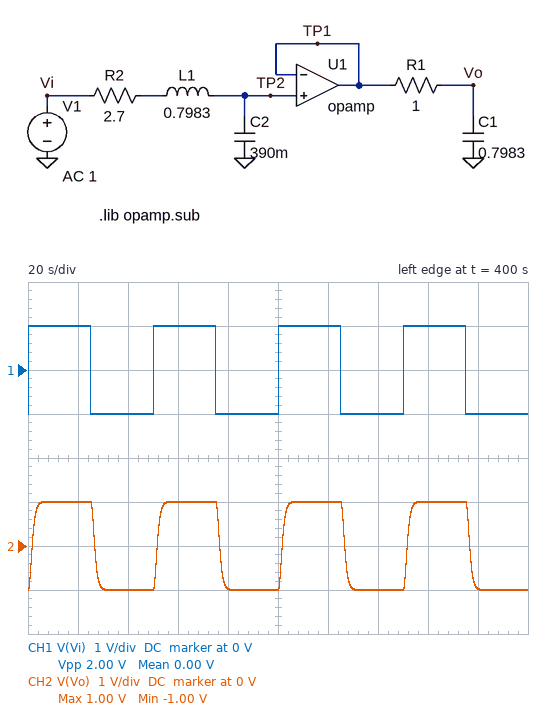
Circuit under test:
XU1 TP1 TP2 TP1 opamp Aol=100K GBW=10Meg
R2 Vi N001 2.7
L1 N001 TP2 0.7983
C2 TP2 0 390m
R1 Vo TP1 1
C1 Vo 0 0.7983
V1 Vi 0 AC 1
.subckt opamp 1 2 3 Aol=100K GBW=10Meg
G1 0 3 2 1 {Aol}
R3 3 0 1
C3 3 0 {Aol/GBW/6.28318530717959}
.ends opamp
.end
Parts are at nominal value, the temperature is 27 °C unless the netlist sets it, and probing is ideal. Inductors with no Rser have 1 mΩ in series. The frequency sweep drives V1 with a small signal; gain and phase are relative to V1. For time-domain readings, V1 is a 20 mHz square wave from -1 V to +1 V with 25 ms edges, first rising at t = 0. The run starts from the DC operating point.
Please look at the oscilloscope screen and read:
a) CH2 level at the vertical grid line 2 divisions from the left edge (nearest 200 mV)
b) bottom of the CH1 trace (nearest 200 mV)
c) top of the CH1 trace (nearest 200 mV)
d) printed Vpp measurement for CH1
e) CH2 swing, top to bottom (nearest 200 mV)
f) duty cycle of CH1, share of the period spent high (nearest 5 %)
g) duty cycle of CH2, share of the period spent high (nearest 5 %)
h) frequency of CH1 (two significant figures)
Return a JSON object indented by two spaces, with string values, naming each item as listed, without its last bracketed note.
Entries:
{
  "CH2 level at the vertical grid line 2 divisions from the left edge": "-1.0 V",
  "bottom of the CH1 trace": "-1.0 V",
  "top of the CH1 trace": "1.0 V",
  "printed Vpp measurement for CH1": "2.00 V",
  "CH2 swing, top to bottom": "2.0 V",
  "duty cycle of CH1, share of the period spent high": "50 %",
  "duty cycle of CH2, share of the period spent high": "50 %",
  "frequency of CH1": "20 mHz"
}
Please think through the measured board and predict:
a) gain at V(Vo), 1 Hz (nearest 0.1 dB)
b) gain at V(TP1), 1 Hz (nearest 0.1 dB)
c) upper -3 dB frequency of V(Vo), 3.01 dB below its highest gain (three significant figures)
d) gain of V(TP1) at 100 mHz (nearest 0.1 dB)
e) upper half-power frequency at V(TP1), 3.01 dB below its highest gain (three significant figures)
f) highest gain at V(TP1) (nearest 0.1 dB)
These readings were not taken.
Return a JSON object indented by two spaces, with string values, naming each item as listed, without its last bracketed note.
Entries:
{
  "gain at V(Vo), 1 Hz": "-36.5 dB",
  "gain at V(TP1), 1 Hz": "-22.3 dB",
  "upper -3 dB frequency of V(Vo), 3.01 dB below its highest gain": "133 mHz",
  "gain of V(TP1) at 100 mHz": "-0.8 dB",
  "upper half-power frequency at V(TP1), 3.01 dB below its highest gain": "199 mHz",
  "highest gain at V(TP1)": "0 dB"
}
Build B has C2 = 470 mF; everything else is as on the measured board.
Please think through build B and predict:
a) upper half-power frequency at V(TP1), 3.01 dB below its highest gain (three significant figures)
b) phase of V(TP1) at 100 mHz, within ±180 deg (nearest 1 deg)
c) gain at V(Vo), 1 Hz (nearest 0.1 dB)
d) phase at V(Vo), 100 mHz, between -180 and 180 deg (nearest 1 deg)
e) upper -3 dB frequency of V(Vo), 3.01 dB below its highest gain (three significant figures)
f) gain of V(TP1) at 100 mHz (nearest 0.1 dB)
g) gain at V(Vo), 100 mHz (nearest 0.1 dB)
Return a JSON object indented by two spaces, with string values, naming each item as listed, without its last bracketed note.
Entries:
{
  "upper half-power frequency at V(TP1), 3.01 dB below its highest gain": "159 mHz",
  "phase of V(TP1) at 100 mHz, within ±180 deg": "-43 deg",
  "gain at V(Vo), 1 Hz": "-38.2 dB",
  "phase at V(Vo), 100 mHz, between -180 and 180 deg": "-70 deg",
  "upper -3 dB frequency of V(Vo), 3.01 dB below its highest gain": "116 mHz",
  "gain of V(TP1) at 100 mHz": "-1.3 dB",
  "gain at V(Vo), 100 mHz": "-2.3 dB"
}
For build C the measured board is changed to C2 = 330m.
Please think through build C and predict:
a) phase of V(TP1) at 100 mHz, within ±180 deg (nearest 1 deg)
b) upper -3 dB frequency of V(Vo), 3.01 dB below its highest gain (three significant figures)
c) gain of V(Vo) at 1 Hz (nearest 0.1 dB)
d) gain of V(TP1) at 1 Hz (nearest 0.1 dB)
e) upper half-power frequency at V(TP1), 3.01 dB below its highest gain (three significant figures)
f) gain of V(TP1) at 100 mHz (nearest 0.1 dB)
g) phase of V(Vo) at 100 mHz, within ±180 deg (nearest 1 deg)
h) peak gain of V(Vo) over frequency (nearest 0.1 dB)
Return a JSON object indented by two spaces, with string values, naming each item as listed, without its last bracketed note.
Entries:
{
  "phase of V(TP1) at 100 mHz, within ±180 deg": "-32 deg",
  "upper -3 dB frequency of V(Vo), 3.01 dB below its highest gain": "149 mHz",
  "gain of V(Vo) at 1 Hz": "-35.0 dB",
  "gain of V(TP1) at 1 Hz": "-20.8 dB",
  "upper half-power frequency at V(TP1), 3.01 dB below its highest gain": "243 mHz",
  "gain of V(TP1) at 100 mHz": "-0.5 dB",
  "phase of V(Vo) at 100 mHz, within ±180 deg": "-59 deg",
  "peak gain of V(Vo) over frequency": "0 dB"
}
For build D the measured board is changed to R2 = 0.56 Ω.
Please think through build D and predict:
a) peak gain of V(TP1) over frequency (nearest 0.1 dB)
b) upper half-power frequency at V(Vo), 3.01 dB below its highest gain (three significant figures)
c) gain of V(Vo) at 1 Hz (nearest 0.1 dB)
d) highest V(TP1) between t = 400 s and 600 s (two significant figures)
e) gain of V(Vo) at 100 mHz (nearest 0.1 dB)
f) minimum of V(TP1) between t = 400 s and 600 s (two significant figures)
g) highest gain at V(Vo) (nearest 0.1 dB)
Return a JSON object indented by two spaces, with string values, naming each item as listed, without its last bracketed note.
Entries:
{
  "peak gain of V(TP1) over frequency": "8.3 dB",
  "upper half-power frequency at V(Vo), 3.01 dB below its highest gain": "316 mHz",
  "gain of V(Vo) at 1 Hz": "-35.3 dB",
  "highest V(TP1) between t = 400 s and 600 s": "2.1 V",
  "gain of V(Vo) at 100 mHz": "0.1 dB",
  "minimum of V(TP1) between t = 400 s and 600 s": "-2.1 V",
  "highest gain at V(Vo)": "3.8 dB"
}
